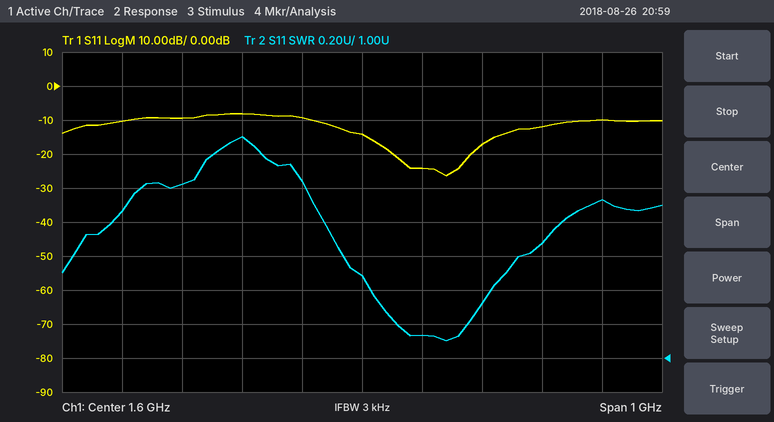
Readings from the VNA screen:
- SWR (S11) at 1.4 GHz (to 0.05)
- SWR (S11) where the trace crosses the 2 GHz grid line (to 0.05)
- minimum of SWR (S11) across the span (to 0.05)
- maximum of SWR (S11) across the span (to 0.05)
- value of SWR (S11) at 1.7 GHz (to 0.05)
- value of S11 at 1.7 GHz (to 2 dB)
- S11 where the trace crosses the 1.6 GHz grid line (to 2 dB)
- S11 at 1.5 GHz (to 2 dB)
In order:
2.30
1.95
1.10
2.30
1.15
-24 dB
-14 dB
-10 dB
